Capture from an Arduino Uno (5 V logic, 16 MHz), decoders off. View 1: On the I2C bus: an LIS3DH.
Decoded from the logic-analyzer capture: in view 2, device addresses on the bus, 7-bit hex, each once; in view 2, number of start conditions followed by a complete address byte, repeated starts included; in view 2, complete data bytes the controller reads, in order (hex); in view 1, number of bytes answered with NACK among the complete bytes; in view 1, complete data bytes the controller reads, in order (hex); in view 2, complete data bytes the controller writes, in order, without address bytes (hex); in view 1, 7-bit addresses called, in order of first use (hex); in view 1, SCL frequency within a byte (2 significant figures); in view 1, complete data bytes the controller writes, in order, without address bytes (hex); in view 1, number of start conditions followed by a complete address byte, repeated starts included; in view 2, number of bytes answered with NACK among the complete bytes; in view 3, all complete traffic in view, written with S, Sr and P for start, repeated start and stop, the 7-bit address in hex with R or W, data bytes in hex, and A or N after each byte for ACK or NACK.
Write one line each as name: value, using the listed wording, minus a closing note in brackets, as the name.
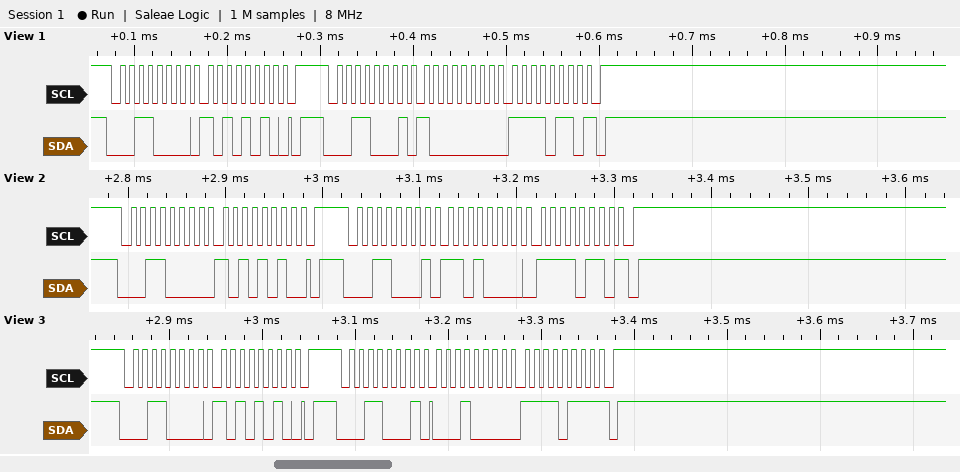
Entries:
in view 2, device addresses on the bus, 7-bit hex, each once: 0x18
in view 2, number of start conditions followed by a complete address byte, repeated starts included: 2
in view 2, complete data bytes the controller reads, in order: D0 F6
in view 1, number of bytes answered with NACK among the complete bytes: 1
in view 1, complete data bytes the controller reads, in order: 80 F6
in view 2, complete data bytes the controller writes, in order, without address bytes: AA
in view 1, 7-bit addresses called, in order of first use: 0x18
in view 1, SCL frequency within a byte: 100 kHz
in view 1, complete data bytes the controller writes, in order, without address bytes: AA
in view 1, number of start conditions followed by a complete address byte, repeated starts included: 2
in view 2, number of bytes answered with NACK among the complete bytes: 1
in view 3, all complete traffic in view, written with S, Sr and P for start, repeated start and stop, the 7-bit address in hex with R or W, data bytes in hex, and A or N after each byte for ACK or NACK: S 18W A AA A P S 18R A 10 A F7 N P
